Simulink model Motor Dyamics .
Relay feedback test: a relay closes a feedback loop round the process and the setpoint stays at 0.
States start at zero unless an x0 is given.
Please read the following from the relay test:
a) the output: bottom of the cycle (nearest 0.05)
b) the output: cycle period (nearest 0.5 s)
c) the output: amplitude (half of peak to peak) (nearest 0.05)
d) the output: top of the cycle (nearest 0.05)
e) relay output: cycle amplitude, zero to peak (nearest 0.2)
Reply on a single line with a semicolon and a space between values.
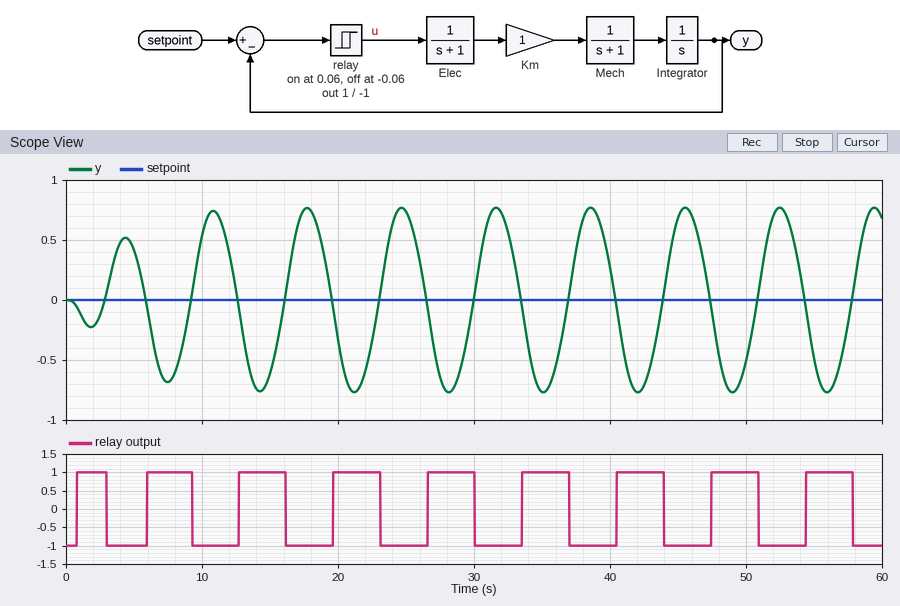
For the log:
-0.75; 7.0 s; 0.75; 0.75; 1.0
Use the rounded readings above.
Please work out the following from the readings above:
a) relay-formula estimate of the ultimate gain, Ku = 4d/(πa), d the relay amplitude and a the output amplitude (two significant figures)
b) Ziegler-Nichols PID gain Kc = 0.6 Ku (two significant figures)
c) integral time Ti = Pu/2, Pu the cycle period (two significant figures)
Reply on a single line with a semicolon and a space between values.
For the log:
1.7; 1.0; 3.5 s
